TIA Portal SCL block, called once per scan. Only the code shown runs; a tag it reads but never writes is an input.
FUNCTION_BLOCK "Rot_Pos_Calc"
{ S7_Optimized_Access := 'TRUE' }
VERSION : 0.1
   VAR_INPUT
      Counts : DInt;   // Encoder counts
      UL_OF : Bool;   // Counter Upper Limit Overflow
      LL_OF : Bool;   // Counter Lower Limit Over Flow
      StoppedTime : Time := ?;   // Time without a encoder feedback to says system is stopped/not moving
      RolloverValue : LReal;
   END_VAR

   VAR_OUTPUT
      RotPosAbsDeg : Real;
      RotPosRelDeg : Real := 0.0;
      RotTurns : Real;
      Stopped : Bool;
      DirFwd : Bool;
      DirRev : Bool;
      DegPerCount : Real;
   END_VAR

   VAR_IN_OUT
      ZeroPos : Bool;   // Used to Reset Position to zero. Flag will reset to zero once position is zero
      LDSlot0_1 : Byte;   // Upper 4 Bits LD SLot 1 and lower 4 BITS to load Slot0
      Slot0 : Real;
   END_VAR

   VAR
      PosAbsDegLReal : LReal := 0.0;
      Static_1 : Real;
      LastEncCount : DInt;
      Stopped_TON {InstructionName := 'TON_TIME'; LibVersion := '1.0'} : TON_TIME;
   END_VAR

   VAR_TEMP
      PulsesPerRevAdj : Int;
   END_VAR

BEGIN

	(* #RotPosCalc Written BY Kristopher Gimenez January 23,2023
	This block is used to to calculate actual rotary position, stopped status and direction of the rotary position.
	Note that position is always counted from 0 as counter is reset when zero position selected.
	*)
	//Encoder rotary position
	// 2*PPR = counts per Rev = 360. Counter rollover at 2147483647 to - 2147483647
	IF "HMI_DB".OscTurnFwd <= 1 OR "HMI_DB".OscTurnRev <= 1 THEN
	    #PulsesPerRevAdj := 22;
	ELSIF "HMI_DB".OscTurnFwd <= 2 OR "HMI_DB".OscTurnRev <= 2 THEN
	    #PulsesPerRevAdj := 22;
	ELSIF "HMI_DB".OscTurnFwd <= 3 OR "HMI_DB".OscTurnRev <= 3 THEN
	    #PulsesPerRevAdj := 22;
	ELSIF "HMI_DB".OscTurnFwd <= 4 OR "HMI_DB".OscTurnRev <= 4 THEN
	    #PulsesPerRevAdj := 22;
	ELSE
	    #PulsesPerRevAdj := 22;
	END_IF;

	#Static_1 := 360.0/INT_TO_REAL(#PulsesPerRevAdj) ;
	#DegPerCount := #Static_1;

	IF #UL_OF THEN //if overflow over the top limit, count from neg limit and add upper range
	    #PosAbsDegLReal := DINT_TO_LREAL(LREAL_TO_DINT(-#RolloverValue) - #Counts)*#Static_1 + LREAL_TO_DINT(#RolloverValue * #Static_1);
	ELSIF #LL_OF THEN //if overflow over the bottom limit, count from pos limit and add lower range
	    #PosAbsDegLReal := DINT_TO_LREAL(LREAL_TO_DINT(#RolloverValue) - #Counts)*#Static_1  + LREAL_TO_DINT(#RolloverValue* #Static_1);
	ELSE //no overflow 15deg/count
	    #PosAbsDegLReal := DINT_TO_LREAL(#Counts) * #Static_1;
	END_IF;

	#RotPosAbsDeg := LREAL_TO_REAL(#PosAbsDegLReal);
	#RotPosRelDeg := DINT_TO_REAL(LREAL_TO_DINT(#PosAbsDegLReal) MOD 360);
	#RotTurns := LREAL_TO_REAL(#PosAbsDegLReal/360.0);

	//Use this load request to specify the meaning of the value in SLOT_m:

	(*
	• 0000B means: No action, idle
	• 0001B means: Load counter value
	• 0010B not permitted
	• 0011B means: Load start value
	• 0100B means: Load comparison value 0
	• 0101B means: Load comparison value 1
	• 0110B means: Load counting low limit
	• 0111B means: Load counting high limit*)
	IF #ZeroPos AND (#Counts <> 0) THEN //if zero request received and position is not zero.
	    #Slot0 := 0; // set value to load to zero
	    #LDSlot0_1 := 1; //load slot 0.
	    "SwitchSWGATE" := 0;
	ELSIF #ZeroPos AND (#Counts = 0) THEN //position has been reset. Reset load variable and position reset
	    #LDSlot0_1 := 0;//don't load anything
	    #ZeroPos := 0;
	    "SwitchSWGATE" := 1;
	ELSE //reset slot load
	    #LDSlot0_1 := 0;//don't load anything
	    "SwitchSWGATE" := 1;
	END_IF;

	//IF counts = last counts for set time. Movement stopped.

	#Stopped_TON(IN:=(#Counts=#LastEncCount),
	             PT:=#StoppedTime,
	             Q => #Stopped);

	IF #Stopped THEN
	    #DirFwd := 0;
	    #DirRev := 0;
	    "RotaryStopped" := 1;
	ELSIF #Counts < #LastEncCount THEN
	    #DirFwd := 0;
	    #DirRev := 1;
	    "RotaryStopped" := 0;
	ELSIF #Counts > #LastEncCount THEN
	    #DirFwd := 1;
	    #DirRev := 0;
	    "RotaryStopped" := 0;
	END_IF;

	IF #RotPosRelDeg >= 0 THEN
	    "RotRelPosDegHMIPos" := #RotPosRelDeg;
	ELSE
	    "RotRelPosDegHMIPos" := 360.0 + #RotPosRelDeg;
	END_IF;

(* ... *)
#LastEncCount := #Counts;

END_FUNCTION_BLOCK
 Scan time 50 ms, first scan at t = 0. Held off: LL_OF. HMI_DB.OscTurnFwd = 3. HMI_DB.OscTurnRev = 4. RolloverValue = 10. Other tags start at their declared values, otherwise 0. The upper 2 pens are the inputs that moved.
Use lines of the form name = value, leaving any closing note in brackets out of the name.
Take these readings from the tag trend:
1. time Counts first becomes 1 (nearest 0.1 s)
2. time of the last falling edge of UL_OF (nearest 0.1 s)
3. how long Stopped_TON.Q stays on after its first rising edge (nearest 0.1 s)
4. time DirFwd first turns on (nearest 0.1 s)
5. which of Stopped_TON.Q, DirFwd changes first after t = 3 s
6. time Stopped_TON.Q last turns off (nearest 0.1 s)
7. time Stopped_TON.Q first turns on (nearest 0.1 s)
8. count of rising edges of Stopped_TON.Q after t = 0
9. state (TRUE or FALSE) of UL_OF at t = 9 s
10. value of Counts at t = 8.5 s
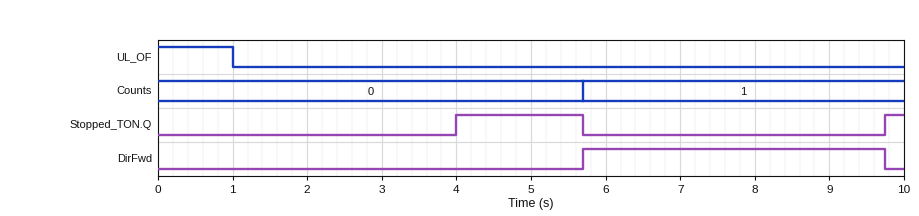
time Counts first becomes 1 = 5.7 s
time of the last falling edge of UL_OF = 1.0 s
how long Stopped_TON.Q stays on after its first rising edge = 1.7 s
time DirFwd first turns on = 5.7 s
which of Stopped_TON.Q, DirFwd changes first after t = 3 s = Stopped_TON.Q
time Stopped_TON.Q last turns off = 5.7 s
time Stopped_TON.Q first turns on = 4.0 s
count of rising edges of Stopped_TON.Q after t = 0 = 2
state (TRUE or FALSE) of UL_OF at t = 9 s = FALSE
value of Counts at t = 8.5 s = 1
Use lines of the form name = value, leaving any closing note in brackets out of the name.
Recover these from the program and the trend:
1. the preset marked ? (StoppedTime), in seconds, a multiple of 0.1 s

the preset marked ? (StoppedTime), in seconds, a multiple of 0.1 s = 4.0 s
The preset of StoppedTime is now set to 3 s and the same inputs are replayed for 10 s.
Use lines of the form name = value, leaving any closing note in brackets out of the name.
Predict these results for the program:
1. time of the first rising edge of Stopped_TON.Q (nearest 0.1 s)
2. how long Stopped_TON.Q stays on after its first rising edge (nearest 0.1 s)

time of the first rising edge of Stopped_TON.Q = 3.0 s
how long Stopped_TON.Q stays on after its first rising edge = 2.7 s
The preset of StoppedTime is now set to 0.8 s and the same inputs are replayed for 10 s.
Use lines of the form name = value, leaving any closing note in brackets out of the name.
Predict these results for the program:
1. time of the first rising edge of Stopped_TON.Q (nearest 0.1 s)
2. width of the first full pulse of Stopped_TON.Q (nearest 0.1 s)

time of the first rising edge of Stopped_TON.Q = 0.8 s
width of the first full pulse of Stopped_TON.Q = 4.9 s
